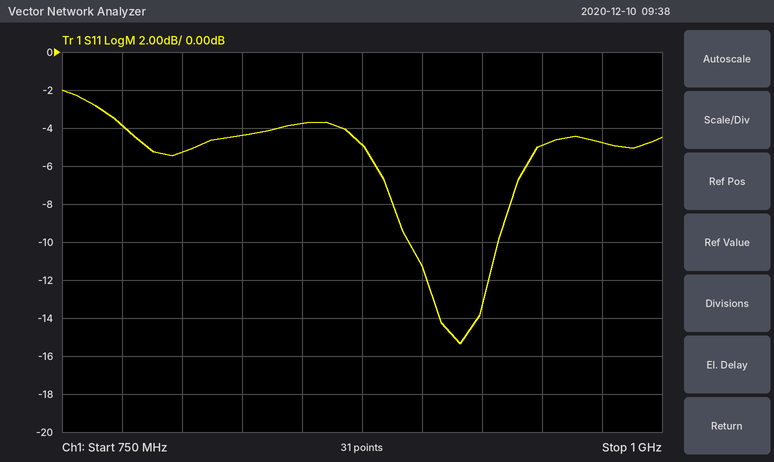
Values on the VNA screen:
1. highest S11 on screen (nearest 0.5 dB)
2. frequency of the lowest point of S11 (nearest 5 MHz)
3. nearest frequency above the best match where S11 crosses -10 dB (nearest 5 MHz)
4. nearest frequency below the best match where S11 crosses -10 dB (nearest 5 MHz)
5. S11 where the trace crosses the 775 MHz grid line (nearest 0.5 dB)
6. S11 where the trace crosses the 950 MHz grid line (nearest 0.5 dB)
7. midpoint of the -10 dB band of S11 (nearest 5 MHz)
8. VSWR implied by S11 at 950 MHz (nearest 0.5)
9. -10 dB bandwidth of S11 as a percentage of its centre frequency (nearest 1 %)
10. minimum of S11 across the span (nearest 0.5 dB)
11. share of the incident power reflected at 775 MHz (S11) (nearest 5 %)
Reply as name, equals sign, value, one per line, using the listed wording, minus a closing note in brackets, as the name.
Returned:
highest S11 on screen = -2.0 dB
frequency of the lowest point of S11 = 915 MHz
nearest frequency above the best match where S11 crosses -10 dB = 930 MHz
nearest frequency below the best match where S11 crosses -10 dB = 895 MHz
S11 where the trace crosses the 775 MHz grid line = -4.0 dB
S11 where the trace crosses the 950 MHz grid line = -5.0 dB
midpoint of the -10 dB band of S11 = 915 MHz
VSWR implied by S11 at 950 MHz = 3.5
-10 dB bandwidth of S11 as a percentage of its centre frequency = 4 %
minimum of S11 across the span = -15.5 dB
share of the incident power reflected at 775 MHz (S11) = 40 %
